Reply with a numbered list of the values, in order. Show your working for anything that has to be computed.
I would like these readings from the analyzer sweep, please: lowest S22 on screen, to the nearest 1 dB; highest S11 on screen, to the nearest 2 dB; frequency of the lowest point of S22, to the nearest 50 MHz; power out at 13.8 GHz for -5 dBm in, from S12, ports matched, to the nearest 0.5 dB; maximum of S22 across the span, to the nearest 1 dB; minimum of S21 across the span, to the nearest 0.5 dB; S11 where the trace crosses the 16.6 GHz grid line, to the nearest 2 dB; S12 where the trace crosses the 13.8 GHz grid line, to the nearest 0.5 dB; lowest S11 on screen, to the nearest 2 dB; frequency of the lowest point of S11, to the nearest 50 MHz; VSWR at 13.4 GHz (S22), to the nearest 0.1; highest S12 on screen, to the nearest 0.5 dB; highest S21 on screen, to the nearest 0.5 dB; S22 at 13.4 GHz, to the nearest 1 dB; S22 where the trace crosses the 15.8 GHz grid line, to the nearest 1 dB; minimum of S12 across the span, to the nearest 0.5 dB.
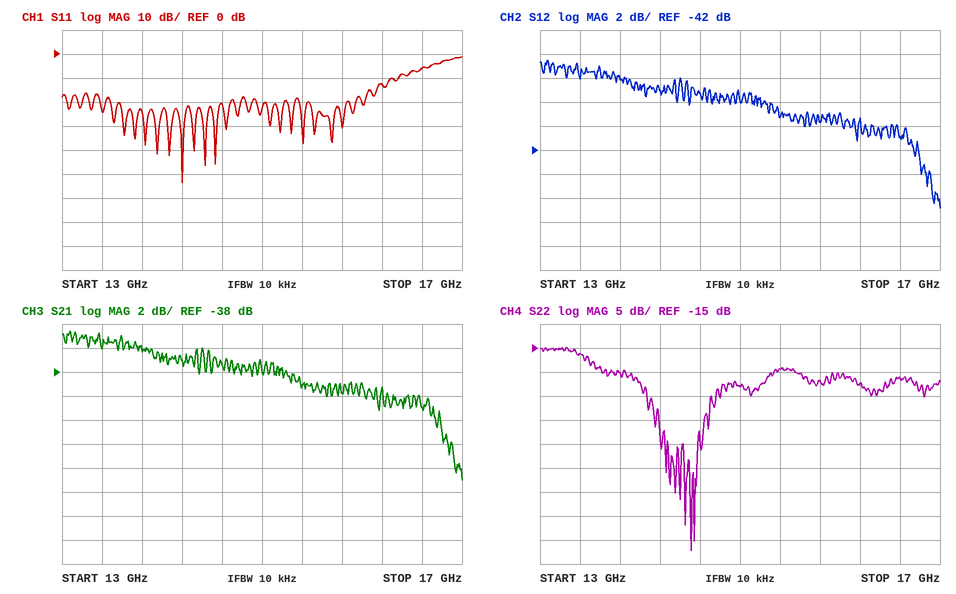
1. -57 dB
2. -2 dB
3. 14.50 GHz
4. -5 dBm + (-36.0 dB) = -41.0 dBm
5. -15 dB
6. -47.0 dB
7. -6 dB
8. -36.0 dB
9. -54 dB
10. 14.20 GHz
11. |Γ| = 10^(-16/20) = 0.1585; VSWR = (1 + 0.1585)/(1 − 0.1585) ≈ 1.4
12. -34.5 dB
13. -34.5 dB
14. -16 dB
15. -22 dB
16. -47.0 dB
